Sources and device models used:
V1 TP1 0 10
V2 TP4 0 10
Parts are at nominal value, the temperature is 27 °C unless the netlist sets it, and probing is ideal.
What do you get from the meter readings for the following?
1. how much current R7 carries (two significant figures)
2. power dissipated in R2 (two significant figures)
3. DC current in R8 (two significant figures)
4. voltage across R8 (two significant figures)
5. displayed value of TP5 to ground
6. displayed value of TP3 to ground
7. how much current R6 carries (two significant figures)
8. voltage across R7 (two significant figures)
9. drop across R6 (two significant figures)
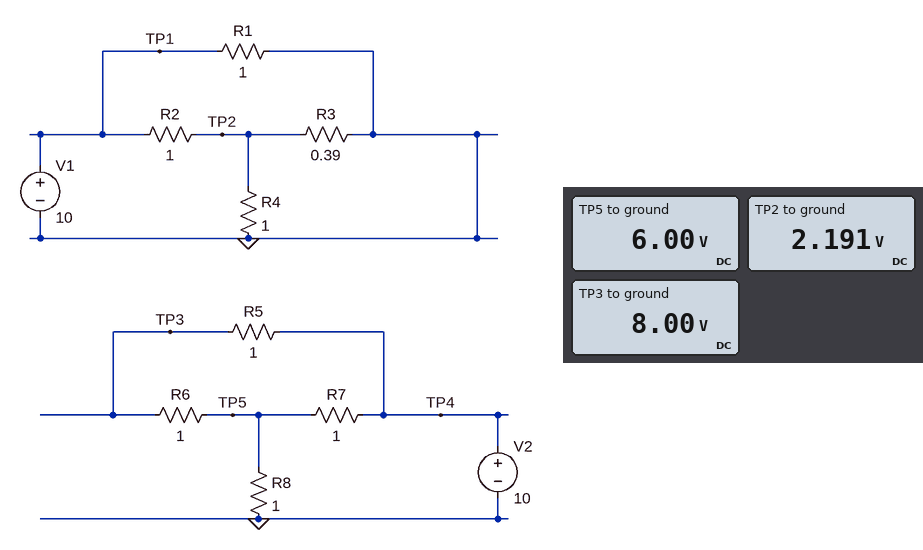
4.0 A
61 W
6.0 A
6.0 V
6.00 V
8.00 V
2.0 A
4.0 V
2.0 V
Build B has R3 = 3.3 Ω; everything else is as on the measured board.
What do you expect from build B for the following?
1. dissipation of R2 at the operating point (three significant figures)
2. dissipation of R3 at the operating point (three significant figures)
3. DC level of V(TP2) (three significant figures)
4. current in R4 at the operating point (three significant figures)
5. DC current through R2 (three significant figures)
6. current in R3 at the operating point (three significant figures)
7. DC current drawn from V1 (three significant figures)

32.0 W
5.71 W
4.34 V
4.34 A
5.66 A
1.32 A
15.7 A
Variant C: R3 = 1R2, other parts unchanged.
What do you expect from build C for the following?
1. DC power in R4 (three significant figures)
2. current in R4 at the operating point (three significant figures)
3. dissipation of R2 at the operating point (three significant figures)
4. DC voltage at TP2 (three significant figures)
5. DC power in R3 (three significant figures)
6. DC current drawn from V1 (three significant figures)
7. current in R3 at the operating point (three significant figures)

12.5 W
3.53 A
41.9 W
3.53 V
10.4 W
16.5 A
2.94 A
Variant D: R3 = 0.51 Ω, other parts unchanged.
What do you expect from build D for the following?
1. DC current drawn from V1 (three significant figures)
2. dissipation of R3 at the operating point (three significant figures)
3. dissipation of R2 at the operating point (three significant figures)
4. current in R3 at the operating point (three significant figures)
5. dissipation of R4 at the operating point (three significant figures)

17.5 A
12.5 W
55.9 W
4.95 A
6.37 W
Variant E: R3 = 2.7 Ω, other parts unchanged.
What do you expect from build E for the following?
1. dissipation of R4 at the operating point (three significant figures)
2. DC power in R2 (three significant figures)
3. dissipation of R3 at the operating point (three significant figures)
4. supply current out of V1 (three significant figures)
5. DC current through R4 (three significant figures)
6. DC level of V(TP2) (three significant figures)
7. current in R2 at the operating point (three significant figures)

17.8 W
33.4 W
6.59 W
15.8 A
4.22 A
4.22 V
5.78 A
